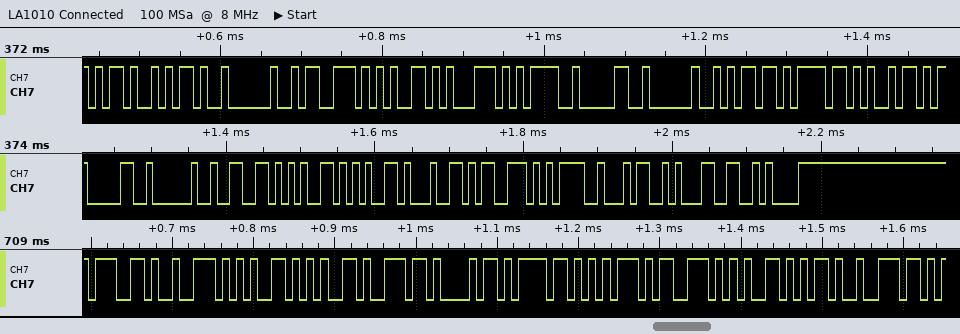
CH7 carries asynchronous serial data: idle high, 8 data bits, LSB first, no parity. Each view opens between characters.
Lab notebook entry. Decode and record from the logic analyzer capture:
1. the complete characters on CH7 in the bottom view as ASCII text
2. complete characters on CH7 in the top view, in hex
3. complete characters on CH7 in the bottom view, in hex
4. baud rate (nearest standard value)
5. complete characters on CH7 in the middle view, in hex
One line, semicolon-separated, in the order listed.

"greenhouse-n"; 2D, 2D, 20, 73, 65, 71, 3D, 30, 20, 6D, 6F, 69; 67, 72, 65, 65, 6E, 68, 6F, 75, 73, 65, 2D, 6E; 115200 baud; 30, 20, 66, 65, 65, 64, 73, 3D, 34, 31, 0A
